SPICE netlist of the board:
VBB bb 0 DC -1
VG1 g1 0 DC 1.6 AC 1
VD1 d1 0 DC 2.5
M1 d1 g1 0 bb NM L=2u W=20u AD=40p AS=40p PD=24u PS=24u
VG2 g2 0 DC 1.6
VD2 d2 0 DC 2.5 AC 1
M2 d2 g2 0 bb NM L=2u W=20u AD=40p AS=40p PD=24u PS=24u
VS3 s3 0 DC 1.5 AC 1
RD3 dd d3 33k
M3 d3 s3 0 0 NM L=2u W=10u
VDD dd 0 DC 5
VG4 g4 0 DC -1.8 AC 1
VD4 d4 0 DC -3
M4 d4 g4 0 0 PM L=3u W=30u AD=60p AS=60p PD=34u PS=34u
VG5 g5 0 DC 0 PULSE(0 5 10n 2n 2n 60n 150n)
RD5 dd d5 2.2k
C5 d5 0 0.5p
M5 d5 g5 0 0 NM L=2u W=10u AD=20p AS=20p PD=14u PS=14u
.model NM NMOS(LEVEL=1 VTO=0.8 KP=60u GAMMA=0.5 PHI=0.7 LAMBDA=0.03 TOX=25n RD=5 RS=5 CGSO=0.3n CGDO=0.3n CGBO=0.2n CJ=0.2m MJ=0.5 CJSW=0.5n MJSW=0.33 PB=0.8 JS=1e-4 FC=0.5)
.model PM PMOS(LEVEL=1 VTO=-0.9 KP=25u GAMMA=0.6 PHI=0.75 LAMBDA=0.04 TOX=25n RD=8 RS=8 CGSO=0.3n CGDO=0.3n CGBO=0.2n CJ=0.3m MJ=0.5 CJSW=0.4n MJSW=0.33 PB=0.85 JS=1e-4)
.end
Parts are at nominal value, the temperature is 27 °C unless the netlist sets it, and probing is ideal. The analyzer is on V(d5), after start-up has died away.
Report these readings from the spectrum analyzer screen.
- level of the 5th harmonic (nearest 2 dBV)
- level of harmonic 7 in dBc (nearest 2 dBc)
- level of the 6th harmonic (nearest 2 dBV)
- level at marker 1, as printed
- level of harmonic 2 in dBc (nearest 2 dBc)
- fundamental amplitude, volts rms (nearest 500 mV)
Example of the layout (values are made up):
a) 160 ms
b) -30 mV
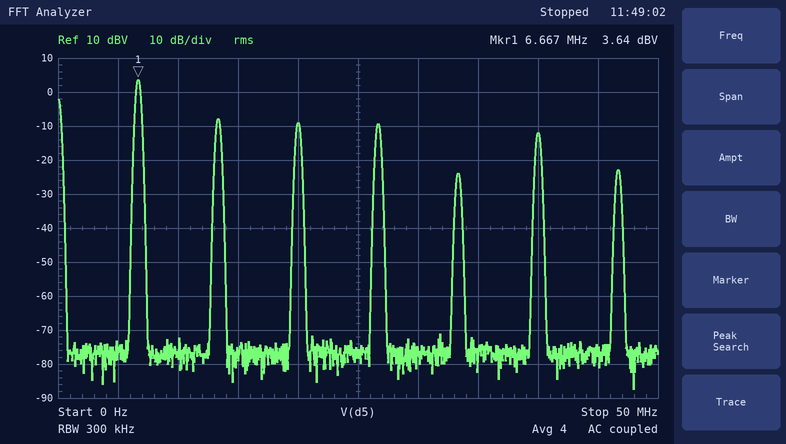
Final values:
a) -24 dBV
b) -26 dBc
c) -12 dBV
d) 3.64 dBV
e) -12 dBc
f) 1.5 V
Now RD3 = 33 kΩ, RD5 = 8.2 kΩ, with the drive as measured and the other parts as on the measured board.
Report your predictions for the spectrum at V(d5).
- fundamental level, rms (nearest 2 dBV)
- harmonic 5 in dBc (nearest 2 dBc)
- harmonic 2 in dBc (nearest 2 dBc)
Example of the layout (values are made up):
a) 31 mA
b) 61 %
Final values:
a) 6 dBV
b) -22 dBc
c) -14 dBc
